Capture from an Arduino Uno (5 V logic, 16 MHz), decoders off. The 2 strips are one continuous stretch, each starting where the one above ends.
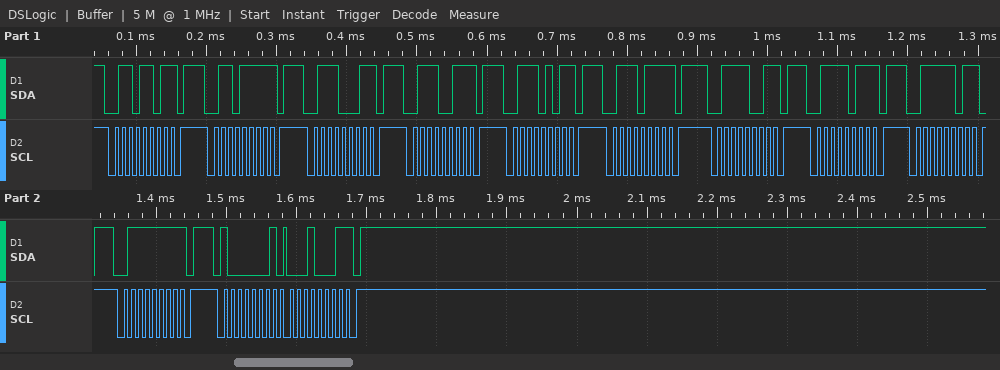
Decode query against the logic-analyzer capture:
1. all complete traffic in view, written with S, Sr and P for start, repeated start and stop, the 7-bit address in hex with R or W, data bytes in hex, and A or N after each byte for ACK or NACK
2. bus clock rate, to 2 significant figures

S 36R N P S 37R N P S 38R N P S 39R N P S 3AR N P S 3BR N P S 3CR N P S 3DR N P S 3ER N P S 3FR N P S 40R A 11 N P
100 kHz
